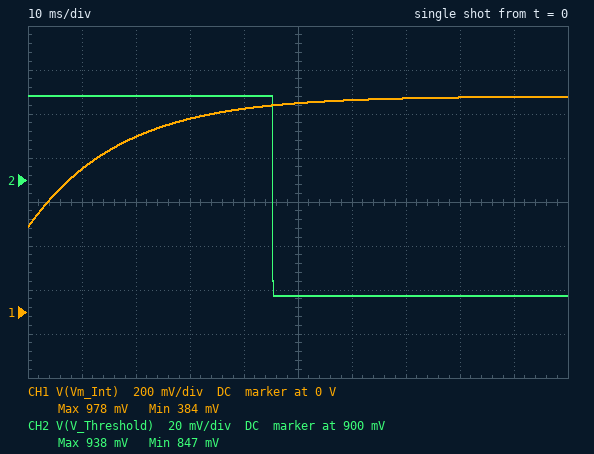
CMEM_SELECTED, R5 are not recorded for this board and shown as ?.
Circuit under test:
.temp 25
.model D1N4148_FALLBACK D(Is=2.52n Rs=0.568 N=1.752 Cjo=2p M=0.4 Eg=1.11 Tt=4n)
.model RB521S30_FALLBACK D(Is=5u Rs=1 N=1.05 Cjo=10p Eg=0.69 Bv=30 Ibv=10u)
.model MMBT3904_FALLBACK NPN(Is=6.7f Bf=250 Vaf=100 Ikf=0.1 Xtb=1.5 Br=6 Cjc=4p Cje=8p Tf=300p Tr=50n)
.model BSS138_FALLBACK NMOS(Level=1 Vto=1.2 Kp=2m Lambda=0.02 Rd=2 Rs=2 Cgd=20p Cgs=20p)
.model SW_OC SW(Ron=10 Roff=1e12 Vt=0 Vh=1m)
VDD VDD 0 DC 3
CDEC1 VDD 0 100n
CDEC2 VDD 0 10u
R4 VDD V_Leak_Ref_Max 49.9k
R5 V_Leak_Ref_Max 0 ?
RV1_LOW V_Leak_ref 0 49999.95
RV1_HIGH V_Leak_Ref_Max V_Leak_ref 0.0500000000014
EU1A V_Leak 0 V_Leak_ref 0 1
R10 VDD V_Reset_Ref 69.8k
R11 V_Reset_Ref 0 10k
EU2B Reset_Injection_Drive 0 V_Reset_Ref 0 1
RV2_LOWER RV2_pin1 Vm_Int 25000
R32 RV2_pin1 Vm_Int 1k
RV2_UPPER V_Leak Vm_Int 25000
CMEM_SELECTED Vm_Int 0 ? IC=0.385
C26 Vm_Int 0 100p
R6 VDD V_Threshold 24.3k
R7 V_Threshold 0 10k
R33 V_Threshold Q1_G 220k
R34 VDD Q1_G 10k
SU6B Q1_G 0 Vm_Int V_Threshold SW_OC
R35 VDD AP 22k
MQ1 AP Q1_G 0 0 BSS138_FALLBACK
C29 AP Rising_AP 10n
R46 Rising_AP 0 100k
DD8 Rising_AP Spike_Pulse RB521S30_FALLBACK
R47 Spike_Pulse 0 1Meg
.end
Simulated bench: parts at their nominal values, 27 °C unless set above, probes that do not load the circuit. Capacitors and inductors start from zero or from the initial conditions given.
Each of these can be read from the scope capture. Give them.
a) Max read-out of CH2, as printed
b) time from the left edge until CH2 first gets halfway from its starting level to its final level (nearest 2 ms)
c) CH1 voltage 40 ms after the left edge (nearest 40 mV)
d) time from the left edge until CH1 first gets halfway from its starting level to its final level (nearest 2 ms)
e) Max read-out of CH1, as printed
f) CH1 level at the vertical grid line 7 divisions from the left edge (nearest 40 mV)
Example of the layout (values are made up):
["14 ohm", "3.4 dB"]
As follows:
["938 mV", "46 ms", "920 mV", "12 ms", "978 mV", "960 mV"]
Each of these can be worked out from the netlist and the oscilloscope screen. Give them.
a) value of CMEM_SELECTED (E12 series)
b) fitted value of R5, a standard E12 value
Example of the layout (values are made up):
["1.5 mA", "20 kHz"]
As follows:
["680 nF", "47 kΩ"]
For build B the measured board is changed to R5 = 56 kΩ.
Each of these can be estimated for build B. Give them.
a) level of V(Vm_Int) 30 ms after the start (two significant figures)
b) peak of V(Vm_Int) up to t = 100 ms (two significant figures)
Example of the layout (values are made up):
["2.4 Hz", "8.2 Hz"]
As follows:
["930 mV", "1.0 V"]
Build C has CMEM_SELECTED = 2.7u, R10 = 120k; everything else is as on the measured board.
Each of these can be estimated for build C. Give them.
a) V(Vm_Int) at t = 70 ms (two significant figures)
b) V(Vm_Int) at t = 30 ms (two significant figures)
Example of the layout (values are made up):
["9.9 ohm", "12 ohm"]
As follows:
["770 mV", "600 mV"]
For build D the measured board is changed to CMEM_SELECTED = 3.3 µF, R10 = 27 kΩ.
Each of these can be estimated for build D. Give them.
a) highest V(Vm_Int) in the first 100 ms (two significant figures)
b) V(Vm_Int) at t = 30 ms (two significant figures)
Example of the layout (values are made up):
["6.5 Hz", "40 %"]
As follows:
["800 mV", "570 mV"]
